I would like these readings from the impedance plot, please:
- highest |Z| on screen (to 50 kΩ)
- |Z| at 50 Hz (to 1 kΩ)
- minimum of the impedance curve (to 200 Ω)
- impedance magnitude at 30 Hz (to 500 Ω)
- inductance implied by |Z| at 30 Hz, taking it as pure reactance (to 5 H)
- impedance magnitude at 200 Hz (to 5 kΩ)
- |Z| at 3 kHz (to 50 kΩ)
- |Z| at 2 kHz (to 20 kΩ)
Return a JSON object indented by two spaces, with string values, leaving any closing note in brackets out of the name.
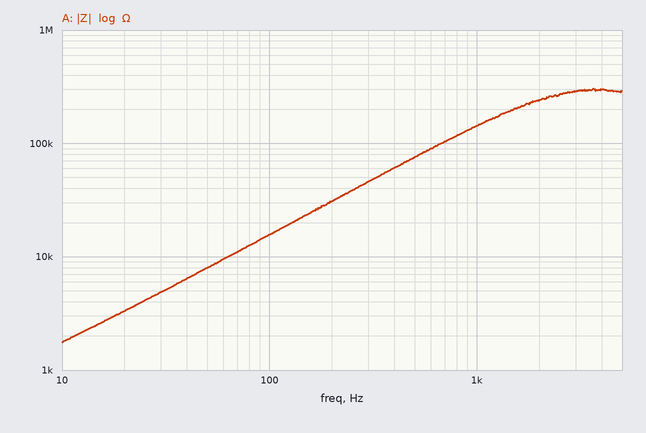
{
  "highest |Z| on screen": "300 kΩ",
  "|Z| at 50 Hz": "8 kΩ",
  "minimum of the impedance curve": "1.8 kΩ",
  "impedance magnitude at 30 Hz": "5.0 kΩ",
  "inductance implied by |Z| at 30 Hz, taking it as pure reactance": "25 H",
  "impedance magnitude at 200 Hz": "30 kΩ",
  "|Z| at 3 kHz": "300 kΩ",
  "|Z| at 2 kHz": "240 kΩ"
}
